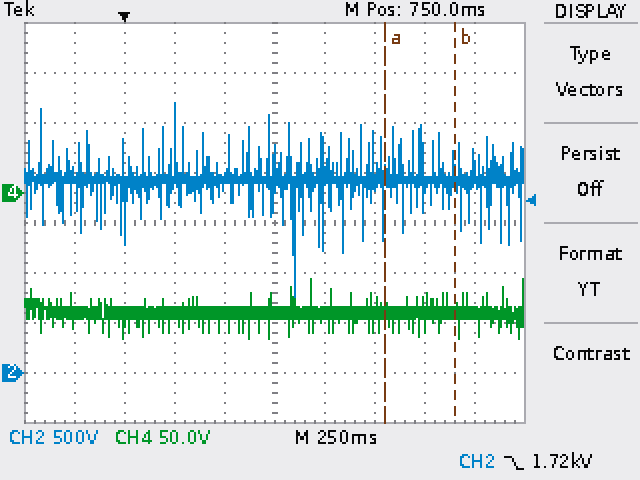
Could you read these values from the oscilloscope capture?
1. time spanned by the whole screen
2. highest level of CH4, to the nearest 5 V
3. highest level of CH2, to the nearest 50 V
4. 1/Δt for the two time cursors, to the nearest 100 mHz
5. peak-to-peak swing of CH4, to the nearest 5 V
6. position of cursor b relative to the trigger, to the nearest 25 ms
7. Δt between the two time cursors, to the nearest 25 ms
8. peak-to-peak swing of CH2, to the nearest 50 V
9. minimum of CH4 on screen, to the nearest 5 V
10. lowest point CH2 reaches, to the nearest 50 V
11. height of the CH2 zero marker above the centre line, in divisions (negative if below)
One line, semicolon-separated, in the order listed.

2.5 s; -85 V; 2.70 kV; 2.9 Hz; 60 V; +1.650 s; 350 ms; 1.95 kV; -145 V; 750 V; -3.0 div
